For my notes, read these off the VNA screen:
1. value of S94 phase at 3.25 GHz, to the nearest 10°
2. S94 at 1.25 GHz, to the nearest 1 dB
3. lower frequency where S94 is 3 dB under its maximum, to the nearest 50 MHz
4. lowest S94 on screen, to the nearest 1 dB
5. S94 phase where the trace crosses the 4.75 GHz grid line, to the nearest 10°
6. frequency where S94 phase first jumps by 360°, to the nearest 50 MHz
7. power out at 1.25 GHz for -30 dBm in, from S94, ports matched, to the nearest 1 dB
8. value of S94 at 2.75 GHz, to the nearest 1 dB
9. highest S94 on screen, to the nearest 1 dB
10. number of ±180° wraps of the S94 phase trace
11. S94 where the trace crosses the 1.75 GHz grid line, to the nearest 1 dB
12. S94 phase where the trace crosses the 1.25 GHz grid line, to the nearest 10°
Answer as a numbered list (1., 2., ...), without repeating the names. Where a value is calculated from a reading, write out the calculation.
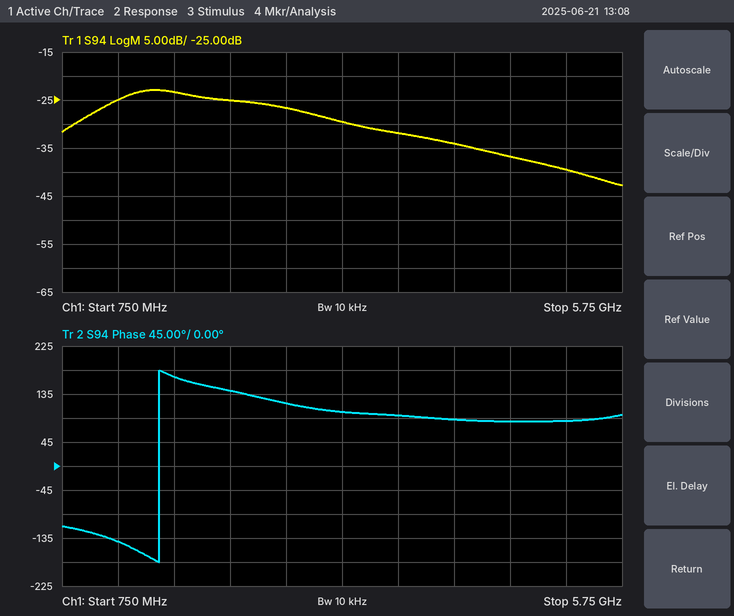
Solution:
1. 100°
2. -25 dB
3. 1.15 GHz
4. -43 dB
5. 80°
6. 1.60 GHz
7. -30 dBm + (-25 dB) = -55 dBm
8. -27 dB
9. -23 dB
10. 1
11. -23 dB
12. -140°
